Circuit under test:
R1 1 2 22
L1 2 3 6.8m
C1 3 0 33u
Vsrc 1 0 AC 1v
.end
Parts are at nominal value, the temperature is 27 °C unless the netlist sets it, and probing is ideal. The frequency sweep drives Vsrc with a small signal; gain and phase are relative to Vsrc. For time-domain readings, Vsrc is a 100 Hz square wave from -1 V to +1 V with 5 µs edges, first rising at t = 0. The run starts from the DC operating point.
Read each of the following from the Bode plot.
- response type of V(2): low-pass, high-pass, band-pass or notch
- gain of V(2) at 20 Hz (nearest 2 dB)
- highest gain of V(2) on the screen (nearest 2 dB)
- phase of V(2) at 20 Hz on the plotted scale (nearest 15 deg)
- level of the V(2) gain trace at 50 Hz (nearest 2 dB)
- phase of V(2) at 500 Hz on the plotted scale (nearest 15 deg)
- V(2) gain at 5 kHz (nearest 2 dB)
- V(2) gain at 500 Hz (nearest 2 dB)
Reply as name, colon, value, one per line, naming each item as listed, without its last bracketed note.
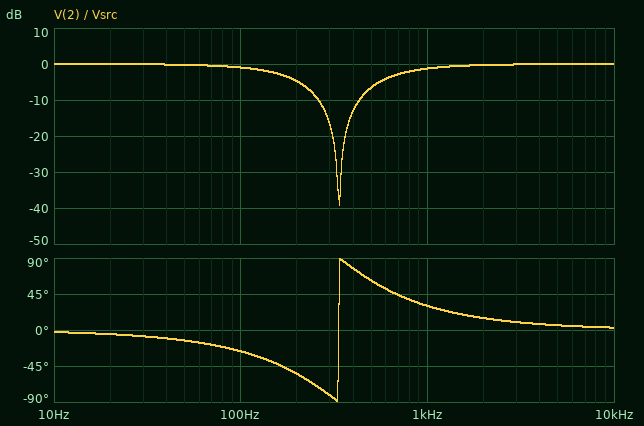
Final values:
response type of V(2): low-pass, high-pass, band-pass or notch: notch
gain of V(2) at 20 Hz: 0 dB
highest gain of V(2) on the screen: 0 dB
phase of V(2) at 20 Hz on the plotted scale: 0 deg
level of the V(2) gain trace at 50 Hz: 0 dB
phase of V(2) at 500 Hz on the plotted scale: 60 deg
V(2) gain at 5 kHz: 0 dB
V(2) gain at 500 Hz: -6 dB
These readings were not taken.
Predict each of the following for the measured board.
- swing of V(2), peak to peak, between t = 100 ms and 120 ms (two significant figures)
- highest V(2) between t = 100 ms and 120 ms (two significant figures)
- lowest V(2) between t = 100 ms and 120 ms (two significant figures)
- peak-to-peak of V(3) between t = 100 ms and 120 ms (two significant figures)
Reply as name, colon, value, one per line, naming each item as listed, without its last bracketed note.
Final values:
swing of V(2), peak to peak, between t = 100 ms and 120 ms: 2.1 V
highest V(2) between t = 100 ms and 120 ms: 1.0 V
lowest V(2) between t = 100 ms and 120 ms: -1.0 V
peak-to-peak of V(3) between t = 100 ms and 120 ms: 2.1 V
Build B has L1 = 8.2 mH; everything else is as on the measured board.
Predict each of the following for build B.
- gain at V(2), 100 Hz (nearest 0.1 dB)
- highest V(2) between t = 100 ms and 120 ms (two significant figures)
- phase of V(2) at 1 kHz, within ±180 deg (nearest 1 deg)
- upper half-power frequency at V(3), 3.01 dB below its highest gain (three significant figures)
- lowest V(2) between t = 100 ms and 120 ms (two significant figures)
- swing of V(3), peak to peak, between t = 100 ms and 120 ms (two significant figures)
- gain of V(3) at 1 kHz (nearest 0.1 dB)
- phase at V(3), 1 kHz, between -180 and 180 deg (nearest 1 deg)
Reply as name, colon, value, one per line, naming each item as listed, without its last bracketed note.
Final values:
gain at V(2), 100 Hz: -1.0 dB
highest V(2) between t = 100 ms and 120 ms: 1.1 V
phase of V(2) at 1 kHz, within ±180 deg: 25 deg
upper half-power frequency at V(3), 3.01 dB below its highest gain: 310 Hz
lowest V(2) between t = 100 ms and 120 ms: -1.1 V
swing of V(3), peak to peak, between t = 100 ms and 120 ms: 2.2 V
gain of V(3) at 1 kHz: -20.6 dB
phase at V(3), 1 kHz, between -180 and 180 deg: -155 deg
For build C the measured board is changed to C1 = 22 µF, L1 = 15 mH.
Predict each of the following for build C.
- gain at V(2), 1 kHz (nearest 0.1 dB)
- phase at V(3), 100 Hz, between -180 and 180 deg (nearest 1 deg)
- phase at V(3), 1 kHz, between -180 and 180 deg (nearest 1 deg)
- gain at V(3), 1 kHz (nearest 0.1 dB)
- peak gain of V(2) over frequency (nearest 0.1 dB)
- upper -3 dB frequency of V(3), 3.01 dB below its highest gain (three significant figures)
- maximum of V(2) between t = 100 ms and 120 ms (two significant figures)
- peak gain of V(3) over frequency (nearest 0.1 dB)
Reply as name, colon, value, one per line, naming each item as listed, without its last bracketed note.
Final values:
gain at V(2), 1 kHz: -0.3 dB
phase at V(3), 100 Hz, between -180 and 180 deg: -19 deg
phase at V(3), 1 kHz, between -180 and 180 deg: -166 deg
gain at V(3), 1 kHz: -21.9 dB
peak gain of V(2) over frequency: 0 dB
upper -3 dB frequency of V(3), 3.01 dB below its highest gain: 329 Hz
maximum of V(2) between t = 100 ms and 120 ms: 1.2 V
peak gain of V(3) over frequency: 2.3 dB
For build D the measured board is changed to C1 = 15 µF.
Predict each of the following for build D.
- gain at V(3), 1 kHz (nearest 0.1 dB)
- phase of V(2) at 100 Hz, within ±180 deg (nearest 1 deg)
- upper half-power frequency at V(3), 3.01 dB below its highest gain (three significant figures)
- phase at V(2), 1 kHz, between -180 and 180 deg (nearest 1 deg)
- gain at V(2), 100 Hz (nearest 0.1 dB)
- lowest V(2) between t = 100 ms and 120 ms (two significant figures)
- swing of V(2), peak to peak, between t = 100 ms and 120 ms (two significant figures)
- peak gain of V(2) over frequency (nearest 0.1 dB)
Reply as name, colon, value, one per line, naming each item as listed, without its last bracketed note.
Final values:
gain at V(3), 1 kHz: -11.3 dB
phase of V(2) at 100 Hz, within ±180 deg: -12 deg
upper half-power frequency at V(3), 3.01 dB below its highest gain: 579 Hz
phase at V(2), 1 kHz, between -180 and 180 deg: 34 deg
gain at V(2), 100 Hz: -0.2 dB
lowest V(2) between t = 100 ms and 120 ms: -1.2 V
swing of V(2), peak to peak, between t = 100 ms and 120 ms: 2.3 V
peak gain of V(2) over frequency: 0 dB
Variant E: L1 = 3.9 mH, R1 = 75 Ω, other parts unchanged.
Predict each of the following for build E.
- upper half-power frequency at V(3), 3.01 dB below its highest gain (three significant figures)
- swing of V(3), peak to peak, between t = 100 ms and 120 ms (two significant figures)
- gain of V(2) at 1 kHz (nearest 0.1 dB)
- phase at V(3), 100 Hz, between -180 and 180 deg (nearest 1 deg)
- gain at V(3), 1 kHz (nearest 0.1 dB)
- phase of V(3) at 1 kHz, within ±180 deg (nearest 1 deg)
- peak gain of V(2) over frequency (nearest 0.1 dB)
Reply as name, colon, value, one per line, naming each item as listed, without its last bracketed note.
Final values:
upper half-power frequency at V(3), 3.01 dB below its highest gain: 65.7 Hz
swing of V(3), peak to peak, between t = 100 ms and 120 ms: 1.5 V
gain of V(2) at 1 kHz: -11.9 dB
phase at V(3), 100 Hz, between -180 and 180 deg: -59 deg
gain at V(3), 1 kHz: -24.1 dB
phase of V(3) at 1 kHz, within ±180 deg: -105 deg
peak gain of V(2) over frequency: 0 dB
